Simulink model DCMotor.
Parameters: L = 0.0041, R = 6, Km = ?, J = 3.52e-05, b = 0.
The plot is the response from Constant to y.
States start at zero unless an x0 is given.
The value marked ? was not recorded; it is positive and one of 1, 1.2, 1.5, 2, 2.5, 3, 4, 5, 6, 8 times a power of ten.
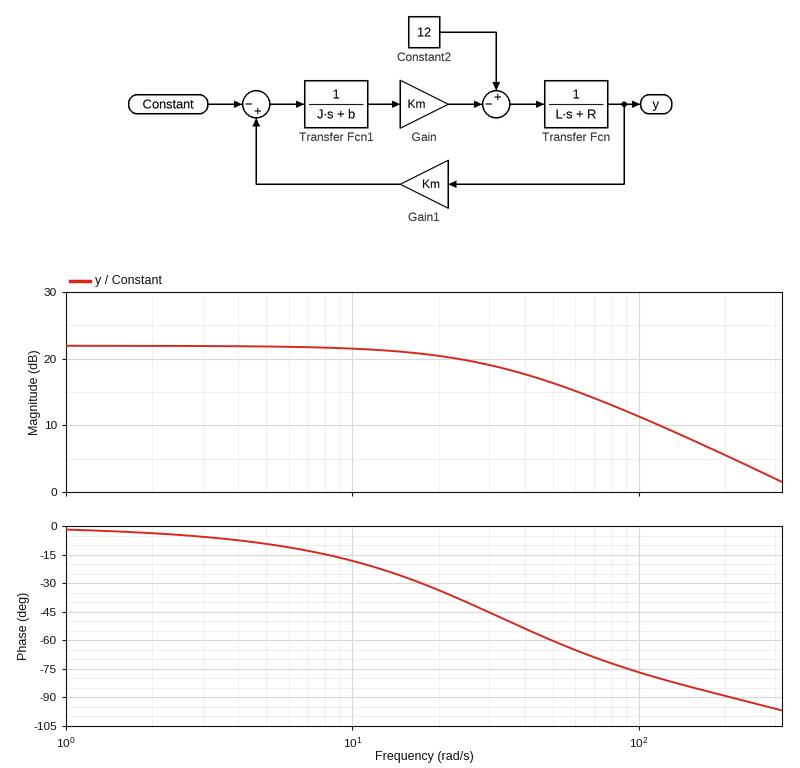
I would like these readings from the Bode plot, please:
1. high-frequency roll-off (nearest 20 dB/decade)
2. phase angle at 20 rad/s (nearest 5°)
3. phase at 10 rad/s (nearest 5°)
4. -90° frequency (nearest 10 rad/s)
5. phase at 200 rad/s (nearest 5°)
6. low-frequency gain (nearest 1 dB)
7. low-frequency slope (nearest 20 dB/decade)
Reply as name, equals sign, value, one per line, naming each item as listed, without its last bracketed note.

high-frequency roll-off = -20 dB/decade
phase angle at 20 rad/s = -35°
phase at 10 rad/s = -20°
-90° frequency = 210 rad/s
phase at 200 rad/s = -90°
low-frequency gain = 22 dB
low-frequency slope = 0 dB/decade
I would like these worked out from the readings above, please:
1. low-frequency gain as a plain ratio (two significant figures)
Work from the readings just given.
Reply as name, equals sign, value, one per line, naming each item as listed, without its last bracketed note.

low-frequency gain as a plain ratio = 13
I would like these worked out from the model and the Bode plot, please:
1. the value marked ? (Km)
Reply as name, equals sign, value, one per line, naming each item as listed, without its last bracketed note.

the value marked ? = 0.08
